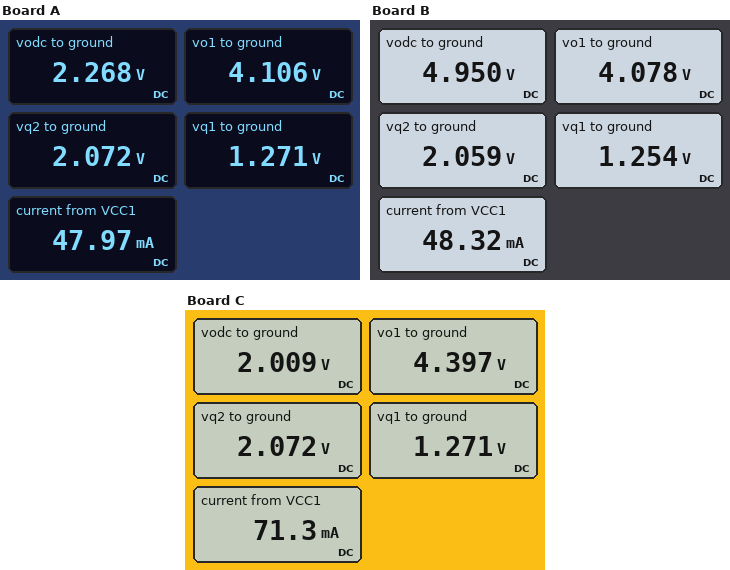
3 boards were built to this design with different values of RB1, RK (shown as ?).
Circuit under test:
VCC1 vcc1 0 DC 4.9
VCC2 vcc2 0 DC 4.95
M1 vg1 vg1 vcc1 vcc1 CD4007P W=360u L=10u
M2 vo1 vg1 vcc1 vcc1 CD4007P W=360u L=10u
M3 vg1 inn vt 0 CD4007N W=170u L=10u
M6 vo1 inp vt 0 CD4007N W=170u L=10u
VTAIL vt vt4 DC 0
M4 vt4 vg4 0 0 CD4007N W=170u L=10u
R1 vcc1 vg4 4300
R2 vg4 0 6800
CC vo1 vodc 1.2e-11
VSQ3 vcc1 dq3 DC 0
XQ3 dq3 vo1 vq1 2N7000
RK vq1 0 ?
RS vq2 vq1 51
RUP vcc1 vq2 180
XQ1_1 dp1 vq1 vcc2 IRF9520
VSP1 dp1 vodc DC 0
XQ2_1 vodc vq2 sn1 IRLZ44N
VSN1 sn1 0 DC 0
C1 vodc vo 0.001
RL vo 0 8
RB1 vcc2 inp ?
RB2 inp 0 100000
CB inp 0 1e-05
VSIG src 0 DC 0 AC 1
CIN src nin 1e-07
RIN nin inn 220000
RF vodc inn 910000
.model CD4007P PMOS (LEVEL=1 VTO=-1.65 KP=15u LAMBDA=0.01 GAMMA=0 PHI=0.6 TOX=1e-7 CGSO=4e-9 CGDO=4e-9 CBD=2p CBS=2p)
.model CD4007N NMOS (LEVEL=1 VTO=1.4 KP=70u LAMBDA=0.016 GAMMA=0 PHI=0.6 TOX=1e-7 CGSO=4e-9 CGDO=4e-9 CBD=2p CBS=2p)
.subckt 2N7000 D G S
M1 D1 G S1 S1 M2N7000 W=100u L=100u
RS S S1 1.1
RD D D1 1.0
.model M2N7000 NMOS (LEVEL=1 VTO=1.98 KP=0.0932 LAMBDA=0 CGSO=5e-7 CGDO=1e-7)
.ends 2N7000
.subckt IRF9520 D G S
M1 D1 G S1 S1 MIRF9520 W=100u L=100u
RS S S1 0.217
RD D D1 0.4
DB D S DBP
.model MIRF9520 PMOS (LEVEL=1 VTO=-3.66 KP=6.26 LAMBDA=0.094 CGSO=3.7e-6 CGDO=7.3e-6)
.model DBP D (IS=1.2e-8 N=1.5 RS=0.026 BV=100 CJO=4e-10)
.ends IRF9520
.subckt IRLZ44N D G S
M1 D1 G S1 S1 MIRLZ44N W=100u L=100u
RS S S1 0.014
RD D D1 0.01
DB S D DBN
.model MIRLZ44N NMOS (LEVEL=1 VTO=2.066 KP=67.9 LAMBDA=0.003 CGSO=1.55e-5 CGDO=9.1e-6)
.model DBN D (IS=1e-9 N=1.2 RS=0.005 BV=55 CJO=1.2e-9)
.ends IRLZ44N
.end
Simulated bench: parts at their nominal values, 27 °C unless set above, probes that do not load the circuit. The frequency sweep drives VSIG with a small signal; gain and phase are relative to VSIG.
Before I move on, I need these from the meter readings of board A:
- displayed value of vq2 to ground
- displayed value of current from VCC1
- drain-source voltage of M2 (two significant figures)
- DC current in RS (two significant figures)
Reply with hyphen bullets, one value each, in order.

- 2.072 V
- 47.97 mA
- -790 mV
- 16 mA
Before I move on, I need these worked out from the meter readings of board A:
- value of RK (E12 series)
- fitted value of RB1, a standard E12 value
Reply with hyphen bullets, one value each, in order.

- 27 Ω
- 120 kΩ
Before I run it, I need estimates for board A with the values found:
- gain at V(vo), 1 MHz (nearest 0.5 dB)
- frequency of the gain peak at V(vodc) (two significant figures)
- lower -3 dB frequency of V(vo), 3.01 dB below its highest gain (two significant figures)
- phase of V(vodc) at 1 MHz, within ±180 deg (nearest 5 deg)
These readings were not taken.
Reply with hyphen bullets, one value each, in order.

- -3.5 dB
- 430 kHz
- 260 kHz
- -25 deg
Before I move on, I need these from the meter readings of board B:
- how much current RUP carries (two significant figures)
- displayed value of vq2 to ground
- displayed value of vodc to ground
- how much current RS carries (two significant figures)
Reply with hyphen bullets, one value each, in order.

- 16 mA
- 2.059 V
- 4.950 V
- 16 mA
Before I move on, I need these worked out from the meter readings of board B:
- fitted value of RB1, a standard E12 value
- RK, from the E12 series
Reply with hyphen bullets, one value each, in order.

- 39 kΩ
- 27 Ω
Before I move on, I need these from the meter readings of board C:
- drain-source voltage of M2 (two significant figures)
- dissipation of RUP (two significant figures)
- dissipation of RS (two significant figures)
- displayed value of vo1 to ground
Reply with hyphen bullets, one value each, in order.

- -500 mV
- 44 mW
- 13 mW
- 4.397 V
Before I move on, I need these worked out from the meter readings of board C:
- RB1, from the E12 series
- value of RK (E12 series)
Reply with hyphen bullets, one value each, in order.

- 150 kΩ
- 18 Ω
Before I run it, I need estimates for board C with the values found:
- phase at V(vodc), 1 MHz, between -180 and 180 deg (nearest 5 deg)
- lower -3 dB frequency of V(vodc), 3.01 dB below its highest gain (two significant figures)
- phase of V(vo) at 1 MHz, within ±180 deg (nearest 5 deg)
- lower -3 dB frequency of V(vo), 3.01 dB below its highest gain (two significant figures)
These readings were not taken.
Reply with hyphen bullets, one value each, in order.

- -20 deg
- 4.8 Hz
- -20 deg
- 19 Hz
